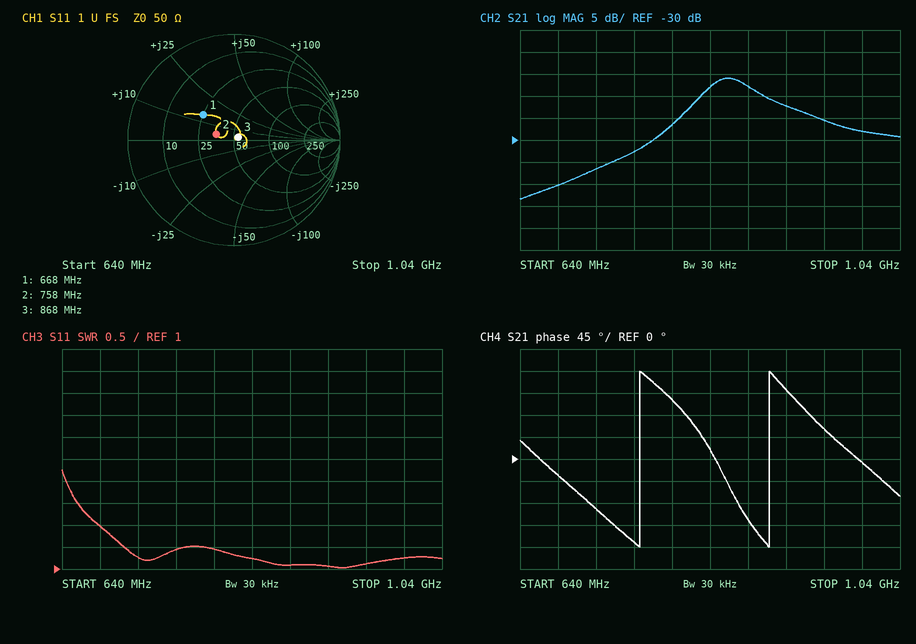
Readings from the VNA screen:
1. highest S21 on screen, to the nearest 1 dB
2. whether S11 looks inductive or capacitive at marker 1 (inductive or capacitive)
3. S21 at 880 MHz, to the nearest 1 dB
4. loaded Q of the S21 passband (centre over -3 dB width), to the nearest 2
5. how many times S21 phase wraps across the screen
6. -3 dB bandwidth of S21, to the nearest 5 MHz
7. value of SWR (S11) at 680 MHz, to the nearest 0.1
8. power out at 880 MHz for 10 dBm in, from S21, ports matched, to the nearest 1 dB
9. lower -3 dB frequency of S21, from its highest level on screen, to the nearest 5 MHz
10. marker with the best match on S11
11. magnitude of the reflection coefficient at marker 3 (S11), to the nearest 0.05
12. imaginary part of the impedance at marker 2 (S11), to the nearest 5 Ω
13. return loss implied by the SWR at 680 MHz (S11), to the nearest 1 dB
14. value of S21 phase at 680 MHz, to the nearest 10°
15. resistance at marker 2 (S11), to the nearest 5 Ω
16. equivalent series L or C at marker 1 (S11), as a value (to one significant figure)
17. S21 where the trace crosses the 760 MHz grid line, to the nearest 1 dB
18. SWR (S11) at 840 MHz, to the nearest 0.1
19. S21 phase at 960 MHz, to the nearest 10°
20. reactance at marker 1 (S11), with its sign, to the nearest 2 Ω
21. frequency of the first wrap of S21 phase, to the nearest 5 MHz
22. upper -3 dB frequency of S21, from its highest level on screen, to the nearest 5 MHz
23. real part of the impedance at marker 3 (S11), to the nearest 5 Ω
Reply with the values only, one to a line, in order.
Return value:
-16 dB
inductive
-18 dB
16
2
55 MHz
2.0
-8 dBm
835 MHz
marker 3
0.05
+5 Ω
10 dB
-30°
35 Ω
3 nH
-33 dB
1.2
60°
+14 Ω
765 MHz
890 MHz
55 Ω
